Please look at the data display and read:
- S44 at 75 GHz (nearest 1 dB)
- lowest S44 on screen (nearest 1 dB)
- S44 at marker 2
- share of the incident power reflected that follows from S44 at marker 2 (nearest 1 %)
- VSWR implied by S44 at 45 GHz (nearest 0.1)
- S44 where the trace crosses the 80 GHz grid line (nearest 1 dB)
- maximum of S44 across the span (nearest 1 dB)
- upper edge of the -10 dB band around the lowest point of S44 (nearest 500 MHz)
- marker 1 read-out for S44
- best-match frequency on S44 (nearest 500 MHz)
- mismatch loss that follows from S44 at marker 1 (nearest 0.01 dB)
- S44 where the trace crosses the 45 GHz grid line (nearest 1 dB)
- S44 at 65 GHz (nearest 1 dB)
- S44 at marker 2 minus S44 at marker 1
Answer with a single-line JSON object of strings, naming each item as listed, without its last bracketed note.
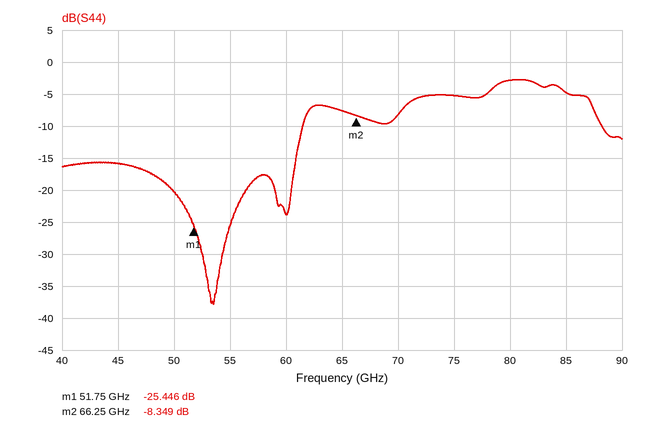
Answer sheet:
{"S44 at 75 GHz": "-5 dB", "lowest S44 on screen": "-38 dB", "S44 at marker 2": "-8.349 dB", "share of the incident power reflected that follows from S44 at marker 2": "15 %", "VSWR implied by S44 at 45 GHz": "1.4", "S44 where the trace crosses the 80 GHz grid line": "-3 dB", "maximum of S44 across the span": "-3 dB", "upper edge of the -10 dB band around the lowest point of S44": "61.5 GHz", "marker 1 read-out for S44": "-25.446 dB", "best-match frequency on S44": "53.5 GHz", "mismatch loss that follows from S44 at marker 1": "0.01 dB", "S44 where the trace crosses the 45 GHz grid line": "-16 dB", "S44 at 65 GHz": "-8 dB", "S44 at marker 2 minus S44 at marker 1": "17.097 dB"}
